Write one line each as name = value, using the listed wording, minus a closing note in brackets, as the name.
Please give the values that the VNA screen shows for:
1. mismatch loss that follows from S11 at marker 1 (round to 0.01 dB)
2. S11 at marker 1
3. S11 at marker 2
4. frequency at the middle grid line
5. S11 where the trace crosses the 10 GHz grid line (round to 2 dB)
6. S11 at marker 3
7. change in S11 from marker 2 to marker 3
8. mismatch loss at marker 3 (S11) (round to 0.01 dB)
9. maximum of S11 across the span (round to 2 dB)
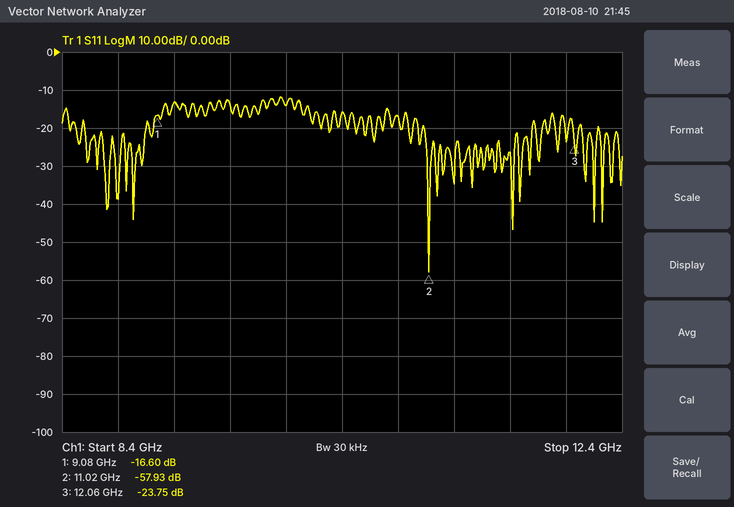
mismatch loss that follows from S11 at marker 1 = 0.10 dB
S11 at marker 1 = -16.60 dB
S11 at marker 2 = -57.93 dB
frequency at the middle grid line = 10.4 GHz
S11 where the trace crosses the 10 GHz grid line = -14 dB
S11 at marker 3 = -23.75 dB
change in S11 from marker 2 to marker 3 = 34.18 dB
mismatch loss at marker 3 (S11) = 0.02 dB
maximum of S11 across the span = -12 dB
